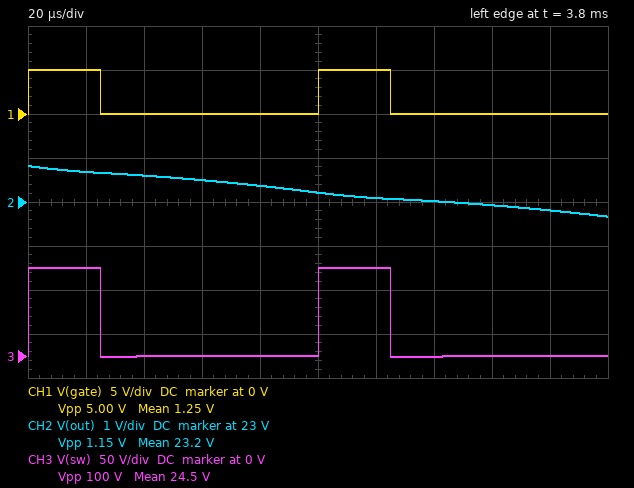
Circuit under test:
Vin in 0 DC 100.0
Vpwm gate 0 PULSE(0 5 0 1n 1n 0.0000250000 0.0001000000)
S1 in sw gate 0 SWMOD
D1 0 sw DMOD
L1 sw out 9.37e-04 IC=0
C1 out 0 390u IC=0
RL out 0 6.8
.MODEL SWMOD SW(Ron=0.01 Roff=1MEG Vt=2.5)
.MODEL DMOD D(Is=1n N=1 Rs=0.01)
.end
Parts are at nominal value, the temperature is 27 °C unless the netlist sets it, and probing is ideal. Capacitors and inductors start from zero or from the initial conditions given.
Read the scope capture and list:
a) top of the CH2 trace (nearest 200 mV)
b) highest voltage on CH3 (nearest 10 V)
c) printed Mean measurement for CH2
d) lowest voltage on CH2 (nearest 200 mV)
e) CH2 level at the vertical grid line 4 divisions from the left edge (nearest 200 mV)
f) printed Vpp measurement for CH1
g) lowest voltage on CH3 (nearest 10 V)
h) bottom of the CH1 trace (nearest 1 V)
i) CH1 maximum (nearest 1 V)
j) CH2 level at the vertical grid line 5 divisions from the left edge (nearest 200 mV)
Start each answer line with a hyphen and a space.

- 23.8 V
- 100 V
- 23.2 V
- 22.6 V
- 23.4 V
- 5.00 V
- 0 V
- 0 V
- 5 V
- 23.2 V
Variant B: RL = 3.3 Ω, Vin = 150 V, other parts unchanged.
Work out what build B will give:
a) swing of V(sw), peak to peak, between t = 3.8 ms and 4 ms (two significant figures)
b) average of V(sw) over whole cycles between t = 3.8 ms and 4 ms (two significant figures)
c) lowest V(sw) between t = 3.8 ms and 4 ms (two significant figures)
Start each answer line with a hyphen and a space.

- 150 V
- 37 V
- -710 mV
